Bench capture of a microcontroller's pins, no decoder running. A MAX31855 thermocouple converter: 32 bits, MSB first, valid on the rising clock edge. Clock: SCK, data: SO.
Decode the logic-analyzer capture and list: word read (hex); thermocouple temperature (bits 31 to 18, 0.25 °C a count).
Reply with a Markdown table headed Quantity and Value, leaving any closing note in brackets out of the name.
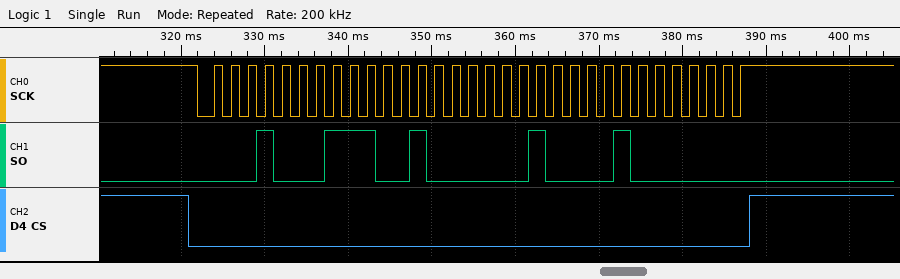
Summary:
| Quantity | Value |
|---|---|
| word read | 0x11C81080 |
| thermocouple temperature | 284.50 °C |
